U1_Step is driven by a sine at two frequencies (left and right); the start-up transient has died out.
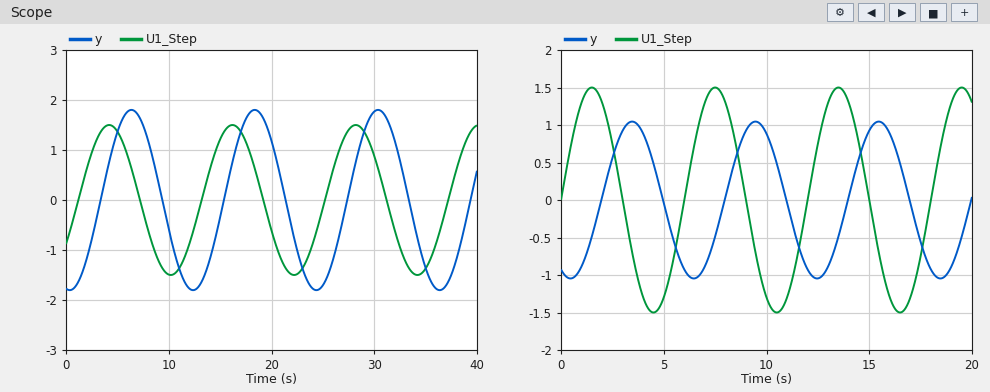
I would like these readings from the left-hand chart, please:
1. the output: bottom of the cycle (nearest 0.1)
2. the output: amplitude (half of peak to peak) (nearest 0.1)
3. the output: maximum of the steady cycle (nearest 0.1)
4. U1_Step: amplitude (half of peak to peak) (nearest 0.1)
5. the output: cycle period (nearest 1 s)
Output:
-1.8
1.8
1.8
1.5
12 s
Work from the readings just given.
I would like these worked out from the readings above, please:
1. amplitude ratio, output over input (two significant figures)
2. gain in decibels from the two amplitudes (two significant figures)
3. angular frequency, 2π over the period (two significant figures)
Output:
1.2
1.6 dB
0.52 rad/s
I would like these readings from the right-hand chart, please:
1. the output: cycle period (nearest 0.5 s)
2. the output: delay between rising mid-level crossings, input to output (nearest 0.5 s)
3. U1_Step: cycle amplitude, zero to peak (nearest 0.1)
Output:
6.0 s
2.0 s
1.5
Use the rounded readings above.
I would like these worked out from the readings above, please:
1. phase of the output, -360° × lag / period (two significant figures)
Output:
-120°
